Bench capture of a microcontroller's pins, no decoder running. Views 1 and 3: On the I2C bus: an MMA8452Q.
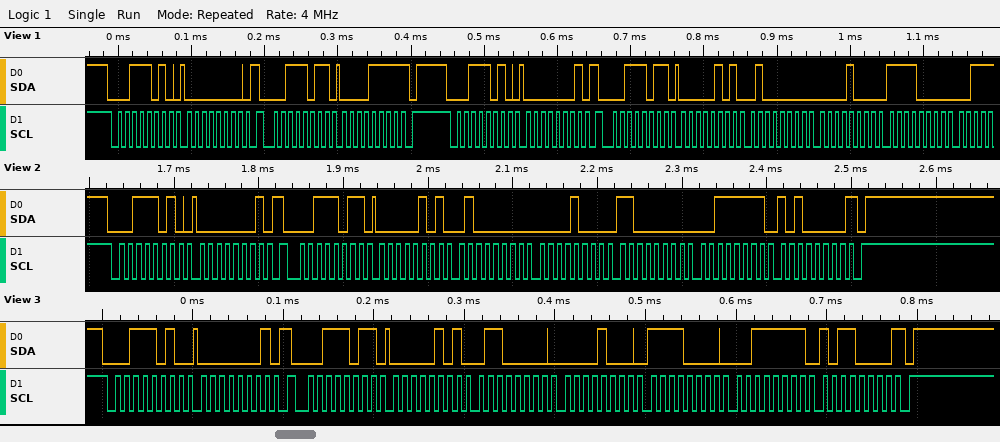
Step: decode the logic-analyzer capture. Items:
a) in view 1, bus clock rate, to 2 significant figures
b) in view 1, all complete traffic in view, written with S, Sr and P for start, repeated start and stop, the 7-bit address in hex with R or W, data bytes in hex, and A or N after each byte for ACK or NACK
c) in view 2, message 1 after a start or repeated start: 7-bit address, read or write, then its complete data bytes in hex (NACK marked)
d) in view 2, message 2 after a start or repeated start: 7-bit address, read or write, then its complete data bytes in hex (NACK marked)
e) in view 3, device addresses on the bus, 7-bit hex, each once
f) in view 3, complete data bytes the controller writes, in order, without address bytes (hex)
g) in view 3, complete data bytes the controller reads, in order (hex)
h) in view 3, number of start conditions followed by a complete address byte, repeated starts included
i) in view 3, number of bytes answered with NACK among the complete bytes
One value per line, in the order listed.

100 kHz
S 1DW A 00 A Sr 1DR A 0F N P S 1DW A 01 A Sr 1DR A 05 A 40 A 08 A F0 A
0x1D write: 01
0x1D read: 05 40 08 C0 3F A0 NACK
0x1D
01
05 60 08 F0 3F B0
2
1
